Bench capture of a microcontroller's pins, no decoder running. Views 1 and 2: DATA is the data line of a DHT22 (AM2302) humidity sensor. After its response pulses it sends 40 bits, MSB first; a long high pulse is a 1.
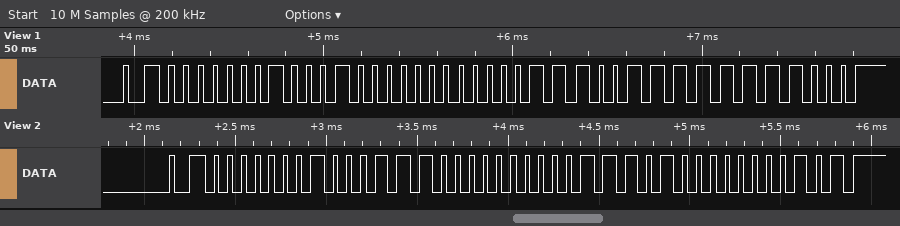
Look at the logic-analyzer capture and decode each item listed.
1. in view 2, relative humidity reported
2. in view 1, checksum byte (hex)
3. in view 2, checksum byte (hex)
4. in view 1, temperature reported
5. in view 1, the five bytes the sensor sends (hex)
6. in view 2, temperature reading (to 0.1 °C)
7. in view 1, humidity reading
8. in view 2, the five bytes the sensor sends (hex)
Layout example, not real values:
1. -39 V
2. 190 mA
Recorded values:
1. 28.4 %
2. 0xF8
3. 0x05
4. 23.1 °C
5. 01 10 00 E7 F8
6. 23.2 °C
7. 27.2 %
8. 01 1C 00 E8 05
